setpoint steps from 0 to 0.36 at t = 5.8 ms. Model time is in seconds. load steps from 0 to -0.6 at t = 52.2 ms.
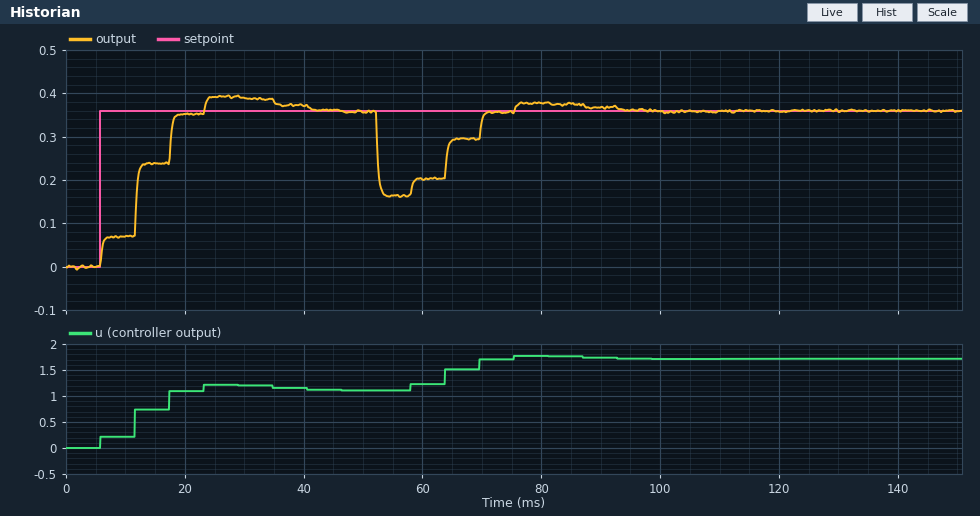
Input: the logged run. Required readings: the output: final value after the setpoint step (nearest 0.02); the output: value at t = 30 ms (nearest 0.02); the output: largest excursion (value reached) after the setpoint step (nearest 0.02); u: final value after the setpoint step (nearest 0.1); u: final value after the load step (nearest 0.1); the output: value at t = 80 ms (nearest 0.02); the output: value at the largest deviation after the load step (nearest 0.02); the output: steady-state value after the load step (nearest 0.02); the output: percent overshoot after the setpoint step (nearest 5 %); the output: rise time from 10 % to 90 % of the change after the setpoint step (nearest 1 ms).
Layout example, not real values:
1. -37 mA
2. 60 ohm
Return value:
1. 0.36
2. 0.38
3. 0.40
4. 1.1
5. 1.7
6. 0.38
7. 0.16
8. 0.36
9. 10 %
10. 12 ms
